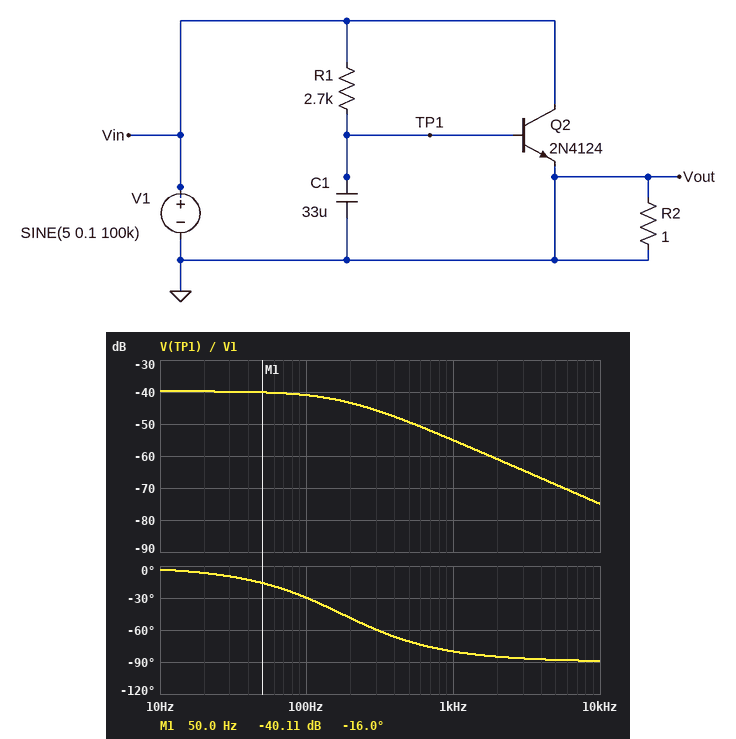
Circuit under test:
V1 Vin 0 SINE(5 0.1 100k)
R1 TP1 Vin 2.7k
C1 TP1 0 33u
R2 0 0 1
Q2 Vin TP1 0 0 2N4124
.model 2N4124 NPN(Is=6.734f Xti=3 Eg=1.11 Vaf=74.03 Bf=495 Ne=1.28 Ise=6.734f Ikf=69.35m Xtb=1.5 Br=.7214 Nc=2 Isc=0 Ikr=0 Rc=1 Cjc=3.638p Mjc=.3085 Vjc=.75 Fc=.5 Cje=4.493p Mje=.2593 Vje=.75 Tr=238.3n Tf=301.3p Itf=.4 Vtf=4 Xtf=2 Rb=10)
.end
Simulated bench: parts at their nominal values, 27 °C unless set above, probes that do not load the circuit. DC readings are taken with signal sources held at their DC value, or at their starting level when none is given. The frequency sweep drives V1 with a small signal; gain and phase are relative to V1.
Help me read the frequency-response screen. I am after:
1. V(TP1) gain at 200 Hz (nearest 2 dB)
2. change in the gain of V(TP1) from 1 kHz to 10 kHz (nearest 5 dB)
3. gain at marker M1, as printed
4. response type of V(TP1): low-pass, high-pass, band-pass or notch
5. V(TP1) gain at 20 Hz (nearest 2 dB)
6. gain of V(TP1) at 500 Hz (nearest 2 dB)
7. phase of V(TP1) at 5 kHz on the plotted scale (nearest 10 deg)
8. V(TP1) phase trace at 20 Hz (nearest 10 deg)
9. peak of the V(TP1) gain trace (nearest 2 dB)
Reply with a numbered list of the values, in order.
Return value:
1. -44 dB
2. -20 dB
3. -40.11 dB
4. low-pass
5. -40 dB
6. -50 dB
7. -90 deg
8. -10 deg
9. -40 dB
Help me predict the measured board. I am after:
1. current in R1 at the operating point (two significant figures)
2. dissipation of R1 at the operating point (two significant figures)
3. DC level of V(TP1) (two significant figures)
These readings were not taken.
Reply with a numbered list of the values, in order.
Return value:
1. 1.5 mA
2. 6.4 mW
3. 840 mV
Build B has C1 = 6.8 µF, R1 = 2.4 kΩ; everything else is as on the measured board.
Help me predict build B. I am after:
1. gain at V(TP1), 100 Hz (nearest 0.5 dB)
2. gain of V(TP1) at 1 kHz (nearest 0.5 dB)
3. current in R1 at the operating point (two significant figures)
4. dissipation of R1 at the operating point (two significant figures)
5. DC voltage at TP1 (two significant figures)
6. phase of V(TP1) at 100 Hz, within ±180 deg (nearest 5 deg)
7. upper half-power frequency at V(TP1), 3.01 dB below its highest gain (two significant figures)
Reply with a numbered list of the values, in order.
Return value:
1. -39.5 dB
2. -43.0 dB
3. 1.7 mA
4. 7.2 mW
5. 850 mV
6. -5 deg
7. 910 Hz
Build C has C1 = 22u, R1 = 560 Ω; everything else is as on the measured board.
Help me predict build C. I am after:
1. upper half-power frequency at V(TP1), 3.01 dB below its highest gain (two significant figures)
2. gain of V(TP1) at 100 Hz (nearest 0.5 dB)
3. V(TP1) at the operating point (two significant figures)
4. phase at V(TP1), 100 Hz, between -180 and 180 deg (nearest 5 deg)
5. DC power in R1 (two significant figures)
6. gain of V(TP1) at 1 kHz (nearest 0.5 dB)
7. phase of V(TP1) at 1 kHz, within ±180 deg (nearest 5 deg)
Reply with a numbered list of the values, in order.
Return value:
1. 540 Hz
2. -32.5 dB
3. 940 mV
4. -10 deg
5. 29 mW
6. -39.0 dB
7. -60 deg
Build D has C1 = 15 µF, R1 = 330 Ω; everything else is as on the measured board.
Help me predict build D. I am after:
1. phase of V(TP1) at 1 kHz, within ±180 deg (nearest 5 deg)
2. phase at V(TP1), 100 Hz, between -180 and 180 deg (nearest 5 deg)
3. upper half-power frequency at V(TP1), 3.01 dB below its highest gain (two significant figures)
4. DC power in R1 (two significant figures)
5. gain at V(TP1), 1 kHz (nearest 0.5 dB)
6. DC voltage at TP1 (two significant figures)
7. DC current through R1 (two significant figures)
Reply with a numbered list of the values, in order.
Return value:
1. -50 deg
2. -5 deg
3. 900 Hz
4. 48 mW
5. -32.5 dB
6. 1.0 V
7. 12 mA
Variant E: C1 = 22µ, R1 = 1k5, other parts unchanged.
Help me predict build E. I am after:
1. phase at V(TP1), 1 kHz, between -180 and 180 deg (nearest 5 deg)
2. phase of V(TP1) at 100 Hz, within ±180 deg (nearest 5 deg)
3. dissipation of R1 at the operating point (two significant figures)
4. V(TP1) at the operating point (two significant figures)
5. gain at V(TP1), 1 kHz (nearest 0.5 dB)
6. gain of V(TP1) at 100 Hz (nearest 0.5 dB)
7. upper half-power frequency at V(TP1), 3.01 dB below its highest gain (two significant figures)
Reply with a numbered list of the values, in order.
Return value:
1. -70 deg
2. -15 deg
3. 11 mW
4. 870 mV
5. -47.0 dB
6. -38.0 dB
7. 370 Hz
